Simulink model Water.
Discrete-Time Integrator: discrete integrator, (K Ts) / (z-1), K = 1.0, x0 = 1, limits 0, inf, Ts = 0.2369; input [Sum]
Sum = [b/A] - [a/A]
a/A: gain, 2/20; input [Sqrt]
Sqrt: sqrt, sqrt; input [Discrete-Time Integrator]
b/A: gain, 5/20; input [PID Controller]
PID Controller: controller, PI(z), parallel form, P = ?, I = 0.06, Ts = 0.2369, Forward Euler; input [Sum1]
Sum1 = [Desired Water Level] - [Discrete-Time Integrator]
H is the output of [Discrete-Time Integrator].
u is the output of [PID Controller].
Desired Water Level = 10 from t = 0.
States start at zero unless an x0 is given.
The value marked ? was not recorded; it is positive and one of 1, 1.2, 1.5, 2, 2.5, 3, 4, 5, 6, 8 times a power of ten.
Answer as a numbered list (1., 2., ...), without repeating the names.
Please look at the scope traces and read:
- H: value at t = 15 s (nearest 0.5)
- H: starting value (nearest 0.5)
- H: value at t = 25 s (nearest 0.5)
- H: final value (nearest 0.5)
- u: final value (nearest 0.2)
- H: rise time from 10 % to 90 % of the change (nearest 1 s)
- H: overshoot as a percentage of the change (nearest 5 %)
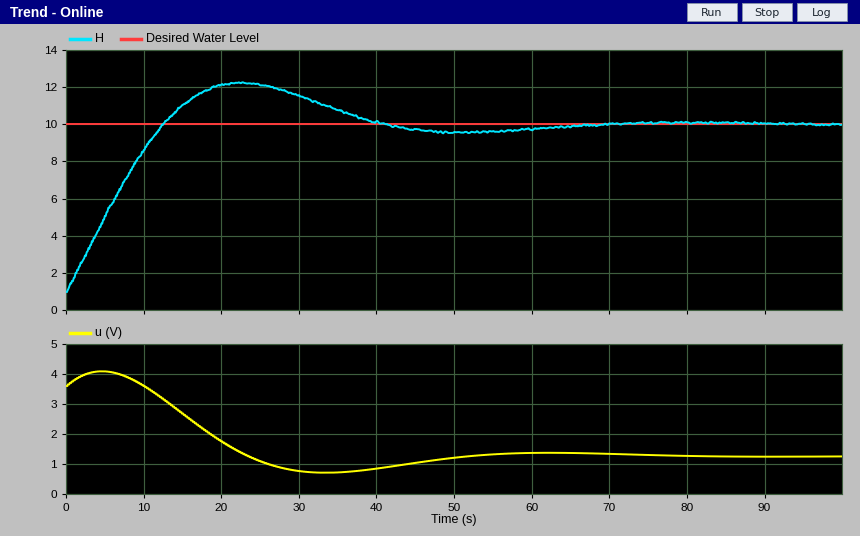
1. 11.0
2. 1.0
3. 12.0
4. 10.0
5. 1.2
6. 10 s
7. 25 %
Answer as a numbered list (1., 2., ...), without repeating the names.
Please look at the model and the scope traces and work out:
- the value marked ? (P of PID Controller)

1. 0.4
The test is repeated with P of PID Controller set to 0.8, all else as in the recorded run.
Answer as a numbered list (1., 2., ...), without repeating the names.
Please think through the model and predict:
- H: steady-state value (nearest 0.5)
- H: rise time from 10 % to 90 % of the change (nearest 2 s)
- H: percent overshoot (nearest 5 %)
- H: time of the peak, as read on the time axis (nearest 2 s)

1. 10.0
2. 8 s
3. 10 %
4. 20 s
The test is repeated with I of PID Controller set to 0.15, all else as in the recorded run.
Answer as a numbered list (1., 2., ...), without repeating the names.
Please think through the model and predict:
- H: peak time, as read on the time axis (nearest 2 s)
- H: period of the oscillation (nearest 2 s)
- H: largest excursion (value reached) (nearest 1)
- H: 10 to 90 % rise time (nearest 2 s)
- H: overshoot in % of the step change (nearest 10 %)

1. 14 s
2. 34 s
3. 14
4. 6 s
5. 40 %
